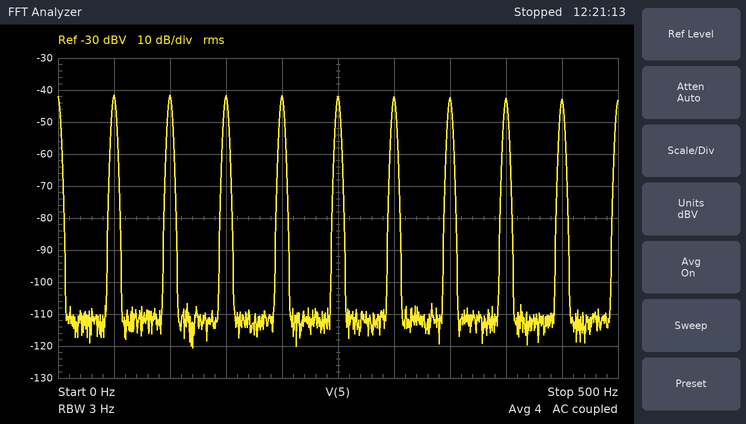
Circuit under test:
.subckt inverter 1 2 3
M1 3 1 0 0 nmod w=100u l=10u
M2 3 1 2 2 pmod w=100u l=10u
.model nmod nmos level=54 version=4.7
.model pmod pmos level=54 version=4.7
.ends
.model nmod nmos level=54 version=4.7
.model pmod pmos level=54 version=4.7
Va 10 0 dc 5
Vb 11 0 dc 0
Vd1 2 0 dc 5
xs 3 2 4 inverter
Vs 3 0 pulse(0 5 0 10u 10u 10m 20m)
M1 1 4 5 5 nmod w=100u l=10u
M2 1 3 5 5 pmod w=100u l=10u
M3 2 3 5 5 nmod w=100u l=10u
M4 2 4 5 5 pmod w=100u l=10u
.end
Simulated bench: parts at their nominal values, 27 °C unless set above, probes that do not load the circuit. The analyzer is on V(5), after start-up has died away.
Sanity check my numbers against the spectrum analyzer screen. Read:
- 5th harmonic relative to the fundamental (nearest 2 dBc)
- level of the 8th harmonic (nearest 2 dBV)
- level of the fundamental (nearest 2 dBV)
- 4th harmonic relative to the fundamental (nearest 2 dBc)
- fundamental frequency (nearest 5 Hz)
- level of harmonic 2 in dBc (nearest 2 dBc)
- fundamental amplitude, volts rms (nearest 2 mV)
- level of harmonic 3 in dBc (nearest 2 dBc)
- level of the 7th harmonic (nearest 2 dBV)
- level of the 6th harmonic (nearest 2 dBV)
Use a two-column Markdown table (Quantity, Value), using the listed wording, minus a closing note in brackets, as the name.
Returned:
| Quantity | Value |
|---|---|
| 5th harmonic relative to the fundamental | 0 dBc |
| level of the 8th harmonic | -42 dBV |
| level of the fundamental | -42 dBV |
| 4th harmonic relative to the fundamental | 0 dBc |
| fundamental frequency | 50 Hz |
| level of harmonic 2 in dBc | 0 dBc |
| fundamental amplitude, volts rms | 8 mV |
| level of harmonic 3 in dBc | 0 dBc |
| level of the 7th harmonic | -42 dBV |
| level of the 6th harmonic | -42 dBV |
